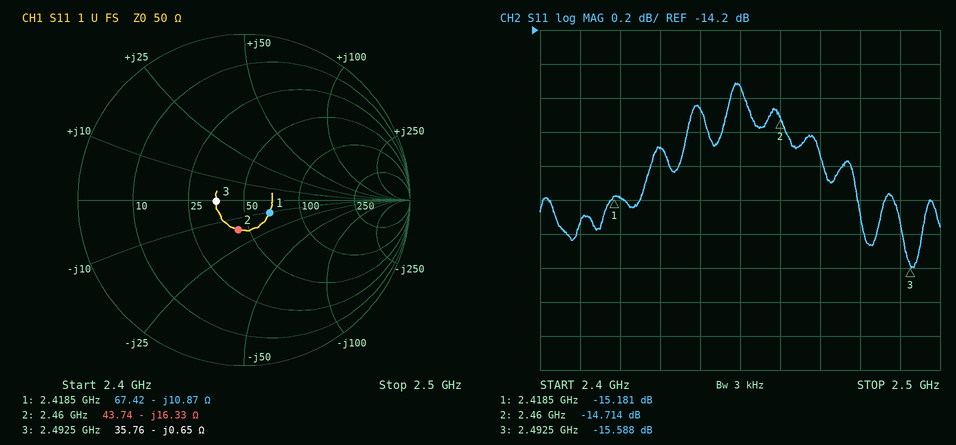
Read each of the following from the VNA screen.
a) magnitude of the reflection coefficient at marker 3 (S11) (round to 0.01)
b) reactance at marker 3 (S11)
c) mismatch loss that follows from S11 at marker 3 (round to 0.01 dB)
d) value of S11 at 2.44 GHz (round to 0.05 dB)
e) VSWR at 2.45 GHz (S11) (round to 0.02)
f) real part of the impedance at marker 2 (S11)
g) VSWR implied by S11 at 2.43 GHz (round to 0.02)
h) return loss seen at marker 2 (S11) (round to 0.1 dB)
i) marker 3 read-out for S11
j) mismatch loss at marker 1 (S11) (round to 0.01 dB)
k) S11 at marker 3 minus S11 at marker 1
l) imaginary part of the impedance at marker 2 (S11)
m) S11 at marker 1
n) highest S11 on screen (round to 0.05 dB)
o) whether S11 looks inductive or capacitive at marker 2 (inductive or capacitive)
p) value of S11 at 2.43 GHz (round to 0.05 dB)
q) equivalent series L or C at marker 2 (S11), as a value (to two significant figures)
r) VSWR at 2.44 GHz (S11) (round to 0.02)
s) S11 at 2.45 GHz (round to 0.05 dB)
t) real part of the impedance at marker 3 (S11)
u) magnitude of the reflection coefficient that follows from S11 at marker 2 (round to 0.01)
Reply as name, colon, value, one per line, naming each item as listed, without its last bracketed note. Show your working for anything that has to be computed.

magnitude of the reflection coefficient at marker 3 (S11): 0.17
reactance at marker 3: -0.65 Ω
mismatch loss that follows from S11 at marker 3: −10 log10(1 − 10^(-15.588/10)) ≈ 0.12 dB
value of S11 at 2.44 GHz: -14.65 dB
VSWR at 2.45 GHz (S11): |Γ| = 10^(-14.55/20) = 0.1873; VSWR = (1 + 0.1873)/(1 − 0.1873) ≈ 1.46
real part of the impedance at marker 2: 43.74 Ω
VSWR implied by S11 at 2.43 GHz: |Γ| = 10^(-14.9/20) = 0.1799; VSWR = (1 + 0.1799)/(1 − 0.1799) ≈ 1.44
return loss seen at marker 2 (S11): 14.7 dB
marker 3 read-out for S11: -15.588 dB
mismatch loss at marker 1 (S11): −10 log10(1 − 10^(-15.181/10)) ≈ 0.13 dB
S11 at marker 3 minus S11 at marker 1: -15.588 − (-15.181) = -0.407 dB
imaginary part of the impedance at marker 2: -16.33 Ω
S11 at marker 1: -15.181 dB
highest S11 on screen: -14.50 dB
whether S11 looks inductive or capacitive at marker 2: capacitive
value of S11 at 2.43 GHz: -14.90 dB
equivalent series L or C at marker 2 (S11), as a value: C = 1/(2π × 2.46 GHz × 16.33 Ω) ≈ 4.0 pF
VSWR at 2.44 GHz (S11): |Γ| = 10^(-14.65/20) = 0.1851; VSWR = (1 + 0.1851)/(1 − 0.1851) ≈ 1.45, so 1.46 to the nearest 0.02
S11 at 2.45 GHz: -14.55 dB
real part of the impedance at marker 3: 35.76 Ω
magnitude of the reflection coefficient that follows from S11 at marker 2: 10^(-14.714/20) ≈ 0.18
